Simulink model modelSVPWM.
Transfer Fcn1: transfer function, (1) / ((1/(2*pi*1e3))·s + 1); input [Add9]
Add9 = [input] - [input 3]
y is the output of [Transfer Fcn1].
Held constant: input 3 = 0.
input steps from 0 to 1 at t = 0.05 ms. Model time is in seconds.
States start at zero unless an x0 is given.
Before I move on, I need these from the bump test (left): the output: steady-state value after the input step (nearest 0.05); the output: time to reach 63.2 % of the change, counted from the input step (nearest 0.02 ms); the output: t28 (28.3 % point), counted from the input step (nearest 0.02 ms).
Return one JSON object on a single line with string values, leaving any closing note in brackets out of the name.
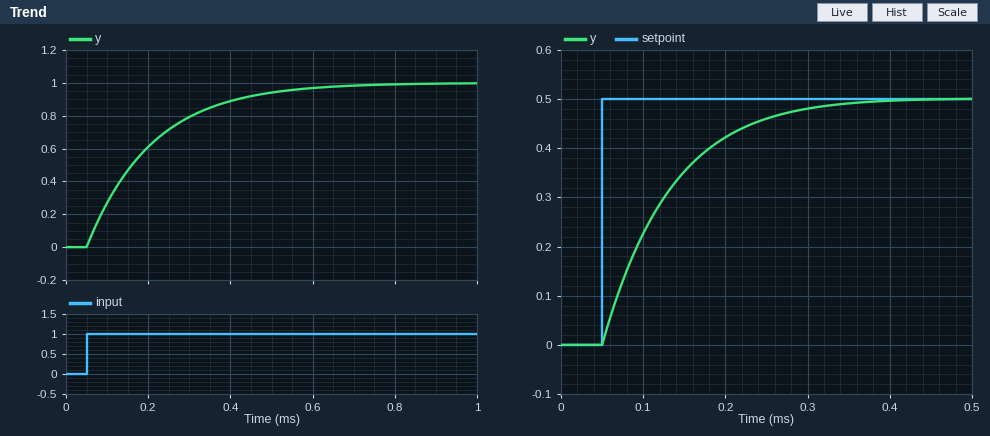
{"the output: steady-state value after the input step": "1.00", "the output: time to reach 63.2 % of the change, counted from the input step": "0.16 ms", "the output: t28 (28.3 % point), counted from the input step": "0.06 ms"}
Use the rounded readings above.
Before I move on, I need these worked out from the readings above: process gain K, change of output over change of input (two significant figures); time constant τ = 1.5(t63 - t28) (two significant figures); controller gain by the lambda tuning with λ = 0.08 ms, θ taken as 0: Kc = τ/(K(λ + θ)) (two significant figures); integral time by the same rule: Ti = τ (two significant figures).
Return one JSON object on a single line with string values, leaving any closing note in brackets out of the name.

{"process gain K, change of output over change of input": "1.0", "time constant τ = 1.5(t63 - t28)": "0.15 ms", "controller gain by the lambda tuning with λ = 0.08 ms, θ taken as 0: Kc = τ/(K(λ + θ))": "1.9", "integral time by the same rule: Ti = τ": "0.15 ms"}
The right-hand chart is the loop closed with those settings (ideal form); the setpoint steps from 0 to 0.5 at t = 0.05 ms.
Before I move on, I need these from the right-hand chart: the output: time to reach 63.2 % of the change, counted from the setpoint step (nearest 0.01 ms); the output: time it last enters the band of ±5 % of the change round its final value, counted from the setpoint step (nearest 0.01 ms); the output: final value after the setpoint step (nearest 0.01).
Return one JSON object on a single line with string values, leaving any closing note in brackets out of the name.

{"the output: time to reach 63.2 % of the change, counted from the setpoint step": "0.08 ms", "the output: time it last enters the band of ±5 % of the change round its final value, counted from the setpoint step": "0.23 ms", "the output: final value after the setpoint step": "0.50"}
